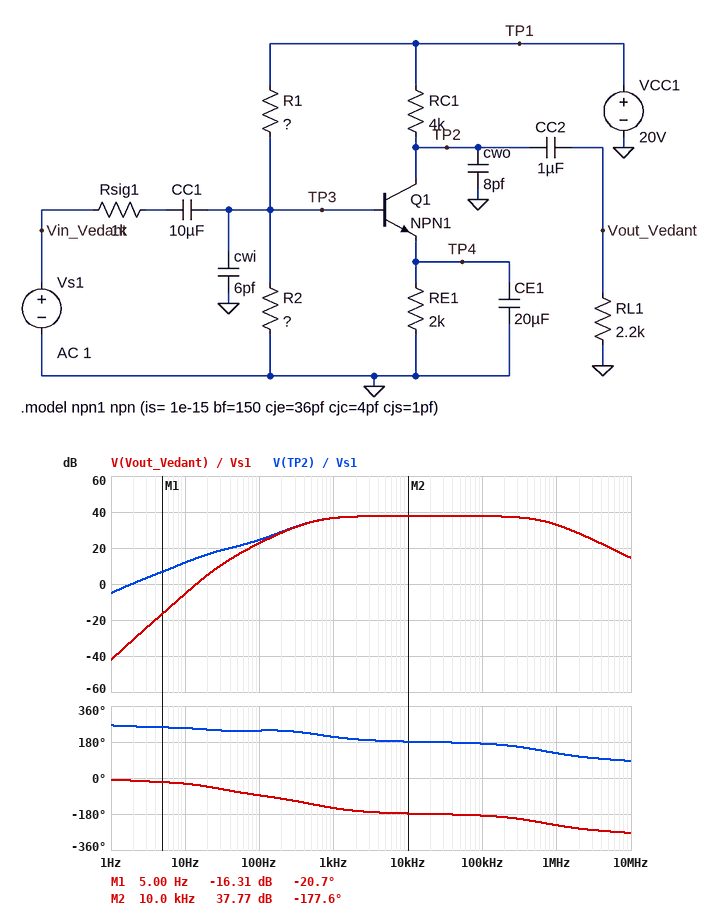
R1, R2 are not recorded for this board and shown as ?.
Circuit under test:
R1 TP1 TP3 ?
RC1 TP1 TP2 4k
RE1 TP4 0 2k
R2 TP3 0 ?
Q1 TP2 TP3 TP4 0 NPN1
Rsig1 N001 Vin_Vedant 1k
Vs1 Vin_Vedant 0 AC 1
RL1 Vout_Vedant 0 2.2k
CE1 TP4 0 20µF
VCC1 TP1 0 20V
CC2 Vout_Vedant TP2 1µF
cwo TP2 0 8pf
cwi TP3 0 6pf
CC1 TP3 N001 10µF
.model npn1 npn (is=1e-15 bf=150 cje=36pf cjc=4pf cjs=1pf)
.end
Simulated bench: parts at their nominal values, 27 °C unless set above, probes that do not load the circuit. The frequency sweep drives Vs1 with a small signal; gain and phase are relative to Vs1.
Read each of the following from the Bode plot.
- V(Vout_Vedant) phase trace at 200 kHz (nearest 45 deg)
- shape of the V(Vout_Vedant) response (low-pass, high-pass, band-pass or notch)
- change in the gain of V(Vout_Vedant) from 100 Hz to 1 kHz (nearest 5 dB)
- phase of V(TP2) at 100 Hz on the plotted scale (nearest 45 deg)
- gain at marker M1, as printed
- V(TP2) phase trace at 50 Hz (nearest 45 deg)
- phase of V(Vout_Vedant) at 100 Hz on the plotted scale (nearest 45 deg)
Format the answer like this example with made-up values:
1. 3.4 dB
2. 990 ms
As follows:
1. -180 deg
2. band-pass
3. 15 dB
4. 225 deg
5. -16.31 dB
6. 225 deg
7. -90 deg
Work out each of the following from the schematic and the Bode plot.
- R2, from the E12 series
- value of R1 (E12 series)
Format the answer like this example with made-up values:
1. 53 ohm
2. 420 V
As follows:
1. 6.8 kΩ
2. 15 kΩ
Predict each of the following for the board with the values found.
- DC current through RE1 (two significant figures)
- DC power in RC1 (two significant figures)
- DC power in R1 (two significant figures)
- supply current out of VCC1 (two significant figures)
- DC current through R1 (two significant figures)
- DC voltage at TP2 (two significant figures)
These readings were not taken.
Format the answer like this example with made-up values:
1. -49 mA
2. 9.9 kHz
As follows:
1. 2.7 mA
2. 29 mW
3. 13 mW
4. 3.6 mA
5. 920 µA
6. 9.2 V
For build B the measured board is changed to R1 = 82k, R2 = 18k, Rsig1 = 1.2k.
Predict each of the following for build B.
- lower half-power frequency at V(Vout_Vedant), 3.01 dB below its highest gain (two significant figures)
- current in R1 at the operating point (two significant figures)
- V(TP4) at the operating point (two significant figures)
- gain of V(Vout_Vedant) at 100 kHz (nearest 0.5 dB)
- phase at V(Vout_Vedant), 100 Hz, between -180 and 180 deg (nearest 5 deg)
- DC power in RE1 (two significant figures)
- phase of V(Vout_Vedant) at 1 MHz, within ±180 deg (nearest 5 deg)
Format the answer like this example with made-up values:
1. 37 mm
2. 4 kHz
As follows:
1. 310 Hz
2. 200 µA
3. 2.7 V
4. 34.0 dB
5. -95 deg
6. 3.8 mW
7. 135 deg
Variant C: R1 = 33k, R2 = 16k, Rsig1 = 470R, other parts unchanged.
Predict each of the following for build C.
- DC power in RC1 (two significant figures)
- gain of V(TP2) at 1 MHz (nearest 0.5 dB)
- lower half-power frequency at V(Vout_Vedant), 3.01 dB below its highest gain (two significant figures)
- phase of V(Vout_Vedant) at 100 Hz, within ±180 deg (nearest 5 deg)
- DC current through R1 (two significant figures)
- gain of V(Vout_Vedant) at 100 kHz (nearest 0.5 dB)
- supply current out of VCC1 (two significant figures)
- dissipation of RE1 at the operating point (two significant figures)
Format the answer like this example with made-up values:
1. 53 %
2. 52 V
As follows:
1. 31 mW
2. 37.5 dB
3. 660 Hz
4. -85 deg
5. 410 µA
6. 41.0 dB
7. 3.2 mA
8. 16 mW
